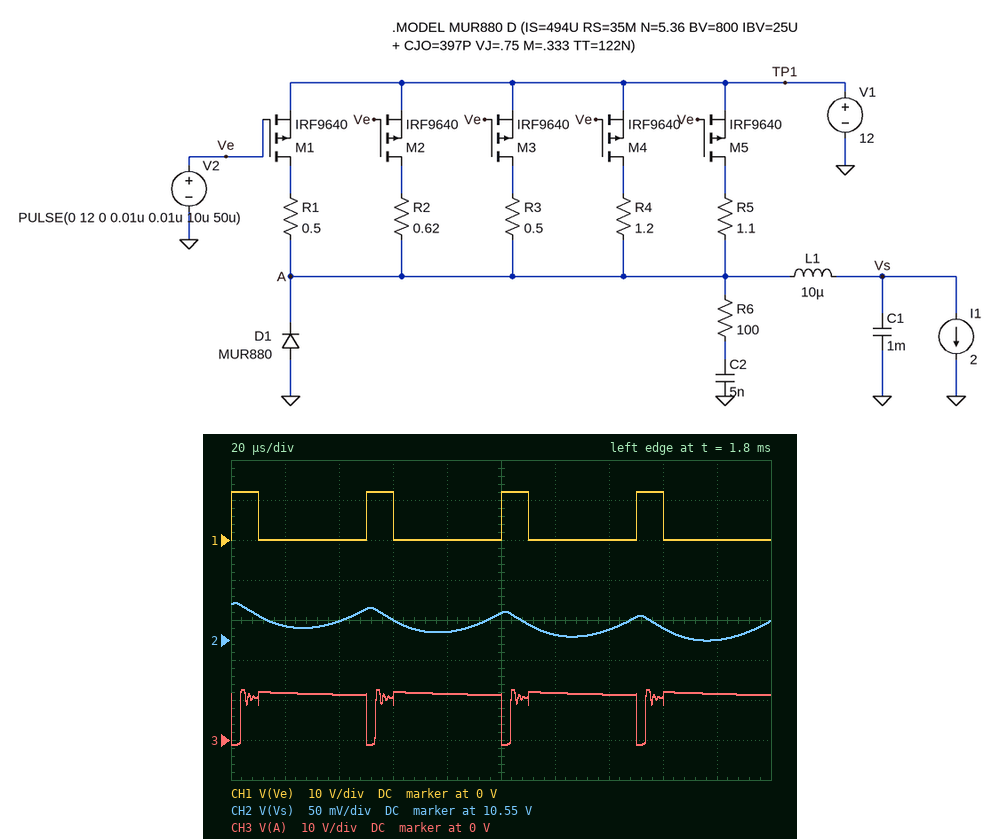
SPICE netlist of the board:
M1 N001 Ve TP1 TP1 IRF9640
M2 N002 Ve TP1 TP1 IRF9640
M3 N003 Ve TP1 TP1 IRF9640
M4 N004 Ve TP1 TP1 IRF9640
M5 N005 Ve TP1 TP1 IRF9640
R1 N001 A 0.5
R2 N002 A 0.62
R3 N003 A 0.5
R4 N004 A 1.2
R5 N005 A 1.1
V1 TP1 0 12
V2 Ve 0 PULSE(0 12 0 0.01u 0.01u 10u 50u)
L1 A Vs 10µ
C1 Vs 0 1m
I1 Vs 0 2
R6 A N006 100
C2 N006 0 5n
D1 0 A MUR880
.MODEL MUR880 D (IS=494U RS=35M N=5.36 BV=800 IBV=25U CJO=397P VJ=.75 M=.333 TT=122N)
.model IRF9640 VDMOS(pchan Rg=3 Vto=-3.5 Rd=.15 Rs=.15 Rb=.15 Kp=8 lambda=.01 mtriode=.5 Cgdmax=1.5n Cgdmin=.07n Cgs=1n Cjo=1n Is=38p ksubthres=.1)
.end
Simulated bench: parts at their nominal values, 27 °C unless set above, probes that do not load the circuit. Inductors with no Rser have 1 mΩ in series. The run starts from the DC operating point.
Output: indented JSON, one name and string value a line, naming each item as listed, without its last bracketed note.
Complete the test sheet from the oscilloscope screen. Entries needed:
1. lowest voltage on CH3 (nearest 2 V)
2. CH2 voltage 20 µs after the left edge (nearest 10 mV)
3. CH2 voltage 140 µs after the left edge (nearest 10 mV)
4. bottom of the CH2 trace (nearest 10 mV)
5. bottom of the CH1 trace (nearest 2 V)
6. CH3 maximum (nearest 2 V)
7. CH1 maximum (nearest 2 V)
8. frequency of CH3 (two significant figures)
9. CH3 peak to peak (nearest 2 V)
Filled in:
{
  "lowest voltage on CH3": "-2 V",
  "CH2 voltage 20 µs after the left edge": "10.57 V",
  "CH2 voltage 140 µs after the left edge": "10.56 V",
  "bottom of the CH2 trace": "10.55 V",
  "bottom of the CH1 trace": "0 V",
  "CH3 maximum": "12 V",
  "CH1 maximum": "12 V",
  "frequency of CH3": "20 kHz",
  "CH3 peak to peak": "14 V"
}
